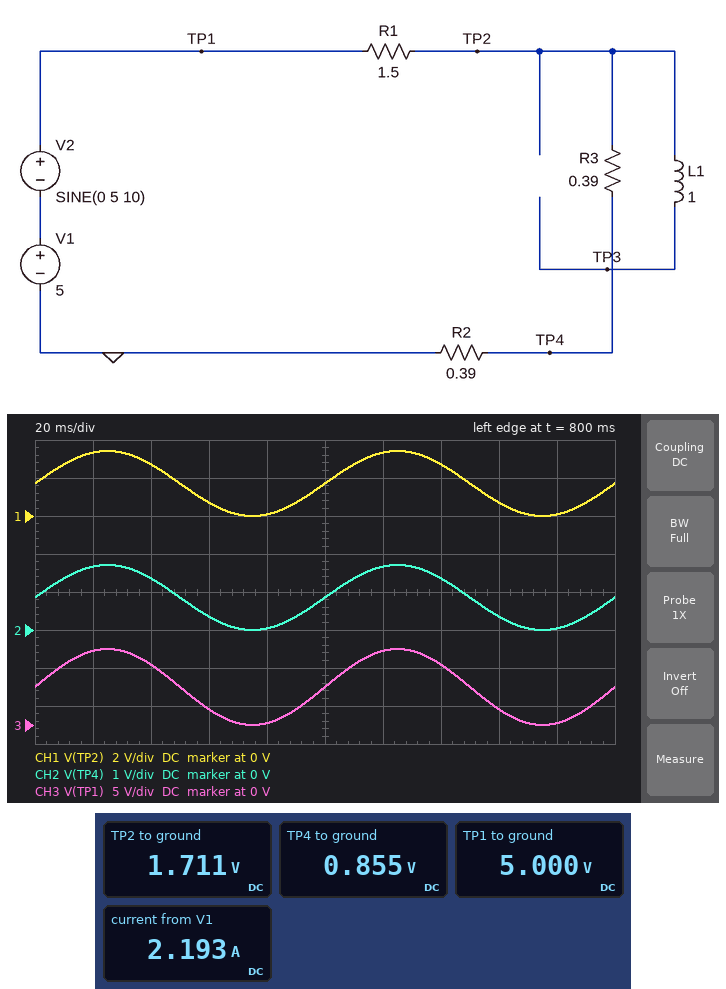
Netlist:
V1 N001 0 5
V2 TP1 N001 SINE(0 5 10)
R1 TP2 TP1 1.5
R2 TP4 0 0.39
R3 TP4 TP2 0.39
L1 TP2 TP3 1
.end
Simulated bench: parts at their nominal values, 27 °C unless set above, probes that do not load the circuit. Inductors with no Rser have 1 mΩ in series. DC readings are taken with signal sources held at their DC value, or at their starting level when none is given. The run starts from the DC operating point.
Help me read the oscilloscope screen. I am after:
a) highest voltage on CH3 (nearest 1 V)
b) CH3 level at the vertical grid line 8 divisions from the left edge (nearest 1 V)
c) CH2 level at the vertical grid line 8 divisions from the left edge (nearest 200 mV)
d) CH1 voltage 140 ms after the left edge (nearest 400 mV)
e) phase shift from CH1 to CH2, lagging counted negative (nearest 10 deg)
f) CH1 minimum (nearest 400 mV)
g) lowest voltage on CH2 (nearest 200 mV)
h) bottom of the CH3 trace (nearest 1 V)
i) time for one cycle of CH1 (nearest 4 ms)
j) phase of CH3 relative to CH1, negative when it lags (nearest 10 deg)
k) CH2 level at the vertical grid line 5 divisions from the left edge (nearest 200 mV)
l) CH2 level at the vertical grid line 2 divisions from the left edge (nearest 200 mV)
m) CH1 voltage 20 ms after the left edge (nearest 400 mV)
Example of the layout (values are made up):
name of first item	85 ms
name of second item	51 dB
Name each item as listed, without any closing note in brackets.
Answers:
highest voltage on CH3	10 V
CH3 level at the vertical grid line 8 divisions from the left edge	2 V
CH2 level at the vertical grid line 8 divisions from the left edge	400 mV
CH1 voltage 140 ms after the left edge	2.8 V
phase shift from CH1 to CH2, lagging counted negative	0 deg
CH1 minimum	0 V
lowest voltage on CH2	0 V
bottom of the CH3 trace	0 V
time for one cycle of CH1	100 ms
phase of CH3 relative to CH1, negative when it lags	0 deg
CH2 level at the vertical grid line 5 divisions from the left edge	800 mV
CH2 level at the vertical grid line 2 divisions from the left edge	1.4 V
CH1 voltage 20 ms after the left edge	3.2 V
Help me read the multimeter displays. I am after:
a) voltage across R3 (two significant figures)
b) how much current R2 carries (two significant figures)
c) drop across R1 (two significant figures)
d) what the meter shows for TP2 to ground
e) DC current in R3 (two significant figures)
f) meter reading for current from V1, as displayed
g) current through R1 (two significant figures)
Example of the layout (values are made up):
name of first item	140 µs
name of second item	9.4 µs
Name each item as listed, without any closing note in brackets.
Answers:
voltage across R3	860 mV
how much current R2 carries	2.2 A
drop across R1	3.3 V
what the meter shows for TP2 to ground	1.711 V
DC current in R3	2.2 A
meter reading for current from V1, as displayed	2.193 A
current through R1	2.2 A
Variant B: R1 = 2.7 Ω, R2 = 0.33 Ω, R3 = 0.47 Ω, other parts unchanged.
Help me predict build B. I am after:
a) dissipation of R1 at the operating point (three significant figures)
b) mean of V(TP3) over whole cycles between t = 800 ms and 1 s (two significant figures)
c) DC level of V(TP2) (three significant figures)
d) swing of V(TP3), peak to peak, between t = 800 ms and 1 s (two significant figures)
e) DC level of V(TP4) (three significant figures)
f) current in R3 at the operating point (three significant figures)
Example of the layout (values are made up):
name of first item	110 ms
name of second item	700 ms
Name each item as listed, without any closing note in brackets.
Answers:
dissipation of R1 at the operating point	5.51 W
mean of V(TP3) over whole cycles between t = 800 ms and 1 s	1.1 V
DC level of V(TP2)	1.14 V
swing of V(TP3), peak to peak, between t = 800 ms and 1 s	2.3 V
DC level of V(TP4)	471 mV
current in R3 at the operating point	1.43 A
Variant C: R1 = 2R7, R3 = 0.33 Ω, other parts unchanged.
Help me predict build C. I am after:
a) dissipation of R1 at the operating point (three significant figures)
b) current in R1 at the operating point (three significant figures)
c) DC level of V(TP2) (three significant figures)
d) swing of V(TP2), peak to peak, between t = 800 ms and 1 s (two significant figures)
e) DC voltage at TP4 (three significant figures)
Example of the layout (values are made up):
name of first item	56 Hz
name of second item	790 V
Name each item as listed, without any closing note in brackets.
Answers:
dissipation of R1 at the operating point	5.77 W
current in R1 at the operating point	1.46 A
DC level of V(TP2)	1.05 V
swing of V(TP2), peak to peak, between t = 800 ms and 1 s	2.1 V
DC voltage at TP4	570 mV
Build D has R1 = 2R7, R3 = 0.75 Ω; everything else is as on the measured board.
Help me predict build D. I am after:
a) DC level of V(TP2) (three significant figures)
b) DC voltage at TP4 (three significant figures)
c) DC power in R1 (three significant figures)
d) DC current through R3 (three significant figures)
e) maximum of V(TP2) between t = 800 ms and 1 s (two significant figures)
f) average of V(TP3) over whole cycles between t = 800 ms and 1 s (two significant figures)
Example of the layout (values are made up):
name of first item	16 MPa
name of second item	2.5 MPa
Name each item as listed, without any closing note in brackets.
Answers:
DC level of V(TP2)	1.48 V
DC voltage at TP4	508 mV
DC power in R1	4.58 W
DC current through R3	1.30 A
maximum of V(TP2) between t = 800 ms and 1 s	3.0 V
average of V(TP3) over whole cycles between t = 800 ms and 1 s	1.5 V
